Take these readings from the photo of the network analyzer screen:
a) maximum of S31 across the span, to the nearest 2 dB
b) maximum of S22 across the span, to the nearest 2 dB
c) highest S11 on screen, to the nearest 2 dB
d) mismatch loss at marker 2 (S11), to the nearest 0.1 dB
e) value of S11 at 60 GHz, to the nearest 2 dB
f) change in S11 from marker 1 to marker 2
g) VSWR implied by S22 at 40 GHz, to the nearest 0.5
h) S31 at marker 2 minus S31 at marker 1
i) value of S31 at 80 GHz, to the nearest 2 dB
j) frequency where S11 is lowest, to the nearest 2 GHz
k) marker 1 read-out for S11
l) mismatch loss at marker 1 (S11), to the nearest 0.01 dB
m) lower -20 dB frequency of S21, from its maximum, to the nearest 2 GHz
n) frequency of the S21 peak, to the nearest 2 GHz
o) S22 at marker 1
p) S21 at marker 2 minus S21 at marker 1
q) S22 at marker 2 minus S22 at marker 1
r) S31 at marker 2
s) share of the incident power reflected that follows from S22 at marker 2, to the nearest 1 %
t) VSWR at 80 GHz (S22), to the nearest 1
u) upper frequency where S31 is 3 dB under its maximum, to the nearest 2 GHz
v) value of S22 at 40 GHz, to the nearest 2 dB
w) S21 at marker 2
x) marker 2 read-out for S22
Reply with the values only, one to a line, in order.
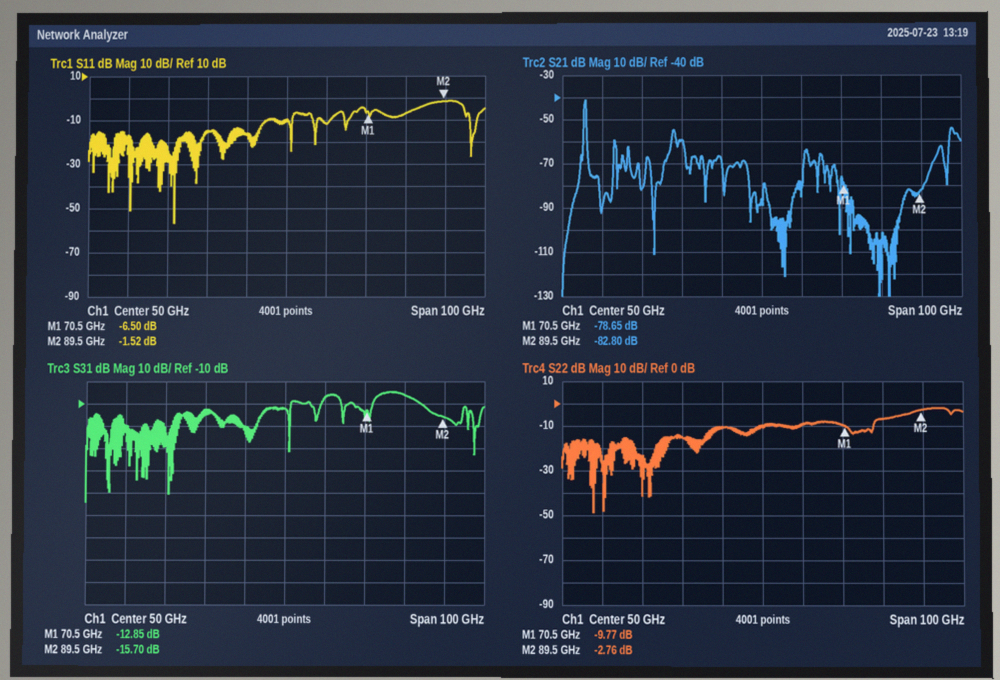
-4 dB
-2 dB
-2 dB
5.3 dB
-12 dB
4.98 dB
2.0
-2.85 dB
-6 dB
22 GHz
-6.50 dB
1.10 dB
6 GHz
6 GHz
-9.77 dB
-4.15 dB
7.01 dB
-15.70 dB
53 %
3
82 GHz
-10 dB
-82.80 dB
-2.76 dB
